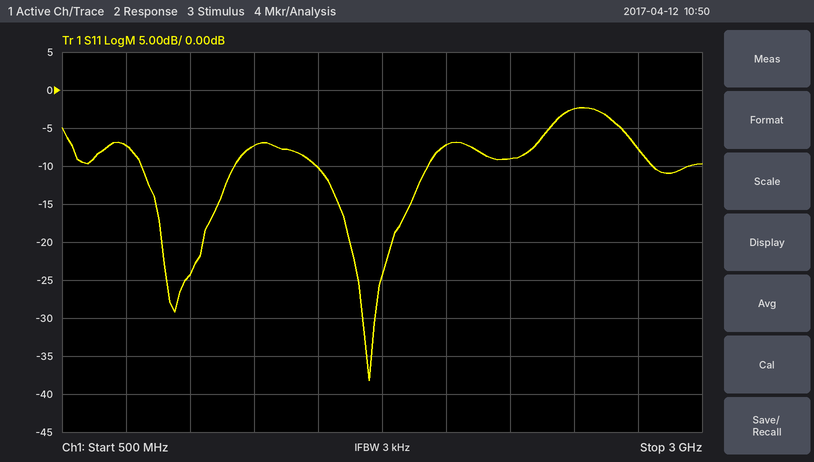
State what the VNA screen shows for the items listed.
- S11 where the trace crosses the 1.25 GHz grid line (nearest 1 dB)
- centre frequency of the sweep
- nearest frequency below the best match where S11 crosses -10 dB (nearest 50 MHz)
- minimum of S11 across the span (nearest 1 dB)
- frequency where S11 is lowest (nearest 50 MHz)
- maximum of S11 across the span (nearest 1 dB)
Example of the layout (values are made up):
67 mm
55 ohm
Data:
-7 dB
1.75 GHz
1.50 GHz
-38 dB
1.70 GHz
-2 dB
